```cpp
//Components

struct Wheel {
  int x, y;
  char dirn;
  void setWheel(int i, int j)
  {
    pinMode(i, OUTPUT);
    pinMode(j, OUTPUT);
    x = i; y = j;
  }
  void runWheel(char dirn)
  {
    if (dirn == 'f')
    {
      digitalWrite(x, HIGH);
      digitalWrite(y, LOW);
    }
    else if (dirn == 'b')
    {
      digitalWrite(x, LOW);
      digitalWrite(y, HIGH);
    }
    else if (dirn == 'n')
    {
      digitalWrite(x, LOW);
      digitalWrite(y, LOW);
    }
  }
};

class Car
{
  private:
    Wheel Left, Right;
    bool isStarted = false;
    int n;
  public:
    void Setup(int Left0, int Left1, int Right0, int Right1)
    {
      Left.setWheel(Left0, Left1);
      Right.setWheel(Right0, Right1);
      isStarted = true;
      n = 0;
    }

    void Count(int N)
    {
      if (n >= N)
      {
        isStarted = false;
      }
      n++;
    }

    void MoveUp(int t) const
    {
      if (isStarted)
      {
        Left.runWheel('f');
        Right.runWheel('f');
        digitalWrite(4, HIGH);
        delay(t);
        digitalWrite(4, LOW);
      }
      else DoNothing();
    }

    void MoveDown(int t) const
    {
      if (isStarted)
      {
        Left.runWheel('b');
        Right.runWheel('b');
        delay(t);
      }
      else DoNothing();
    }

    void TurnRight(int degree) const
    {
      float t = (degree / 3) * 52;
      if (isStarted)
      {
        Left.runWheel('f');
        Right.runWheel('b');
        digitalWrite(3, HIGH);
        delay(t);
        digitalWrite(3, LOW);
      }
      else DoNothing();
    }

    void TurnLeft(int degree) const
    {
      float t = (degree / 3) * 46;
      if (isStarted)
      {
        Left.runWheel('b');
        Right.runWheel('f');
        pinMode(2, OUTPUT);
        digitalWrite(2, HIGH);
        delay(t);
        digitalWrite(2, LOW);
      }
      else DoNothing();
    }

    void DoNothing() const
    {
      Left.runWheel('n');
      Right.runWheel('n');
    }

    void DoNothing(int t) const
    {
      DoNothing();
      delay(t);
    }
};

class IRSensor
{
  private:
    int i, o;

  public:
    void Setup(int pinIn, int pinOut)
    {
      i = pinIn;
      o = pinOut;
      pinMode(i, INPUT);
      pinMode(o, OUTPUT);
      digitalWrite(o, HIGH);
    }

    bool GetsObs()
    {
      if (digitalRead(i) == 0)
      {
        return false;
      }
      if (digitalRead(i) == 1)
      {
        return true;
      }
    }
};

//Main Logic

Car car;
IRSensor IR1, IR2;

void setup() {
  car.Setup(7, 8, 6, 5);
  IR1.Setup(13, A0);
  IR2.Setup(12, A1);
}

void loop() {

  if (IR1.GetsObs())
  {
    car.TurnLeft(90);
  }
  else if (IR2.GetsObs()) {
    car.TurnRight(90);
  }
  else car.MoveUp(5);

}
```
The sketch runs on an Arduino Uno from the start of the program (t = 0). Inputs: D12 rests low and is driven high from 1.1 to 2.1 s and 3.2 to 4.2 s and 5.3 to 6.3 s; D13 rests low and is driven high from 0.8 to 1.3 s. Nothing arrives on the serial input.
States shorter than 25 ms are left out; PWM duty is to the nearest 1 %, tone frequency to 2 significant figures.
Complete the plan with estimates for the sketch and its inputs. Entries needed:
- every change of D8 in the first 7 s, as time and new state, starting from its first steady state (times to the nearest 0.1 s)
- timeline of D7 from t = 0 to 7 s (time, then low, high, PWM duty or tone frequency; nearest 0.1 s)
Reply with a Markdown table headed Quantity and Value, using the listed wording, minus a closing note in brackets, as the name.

| Quantity | Value |
|---|---|
| every change of D8 in the first 7 s, as time and new state, starting from its first steady state | 0 s low; 0.8 s high; 2.2 s low |
| timeline of D7 from t = 0 to 7 s | 0 s high; 0.8 s low; 2.2 s high |
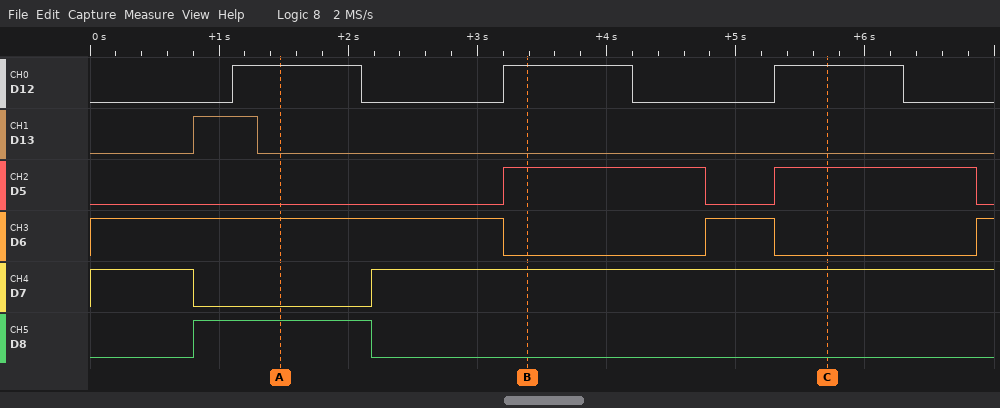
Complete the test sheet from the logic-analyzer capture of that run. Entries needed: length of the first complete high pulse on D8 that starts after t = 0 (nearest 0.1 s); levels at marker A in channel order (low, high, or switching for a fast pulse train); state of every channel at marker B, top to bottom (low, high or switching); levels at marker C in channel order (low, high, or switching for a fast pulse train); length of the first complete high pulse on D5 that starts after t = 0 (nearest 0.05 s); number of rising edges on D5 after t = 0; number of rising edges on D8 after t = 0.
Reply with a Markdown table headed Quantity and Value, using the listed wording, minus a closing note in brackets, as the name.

| Quantity | Value |
|---|---|
| length of the first complete high pulse on D8 that starts after t = 0 | 1.4 s |
| levels at marker A in channel order | D12 high, D13 low, D5 low, D6 high, D7 low, D8 high |
| state of every channel at marker B, top to bottom | D12 high, D13 low, D5 high, D6 low, D7 high, D8 low |
| levels at marker C in channel order | D12 high, D13 low, D5 high, D6 low, D7 high, D8 low |
| length of the first complete high pulse on D5 that starts after t = 0 | 1.55 s |
| number of rising edges on D5 after t = 0 | 2 |
| number of rising edges on D8 after t = 0 | 1 |
